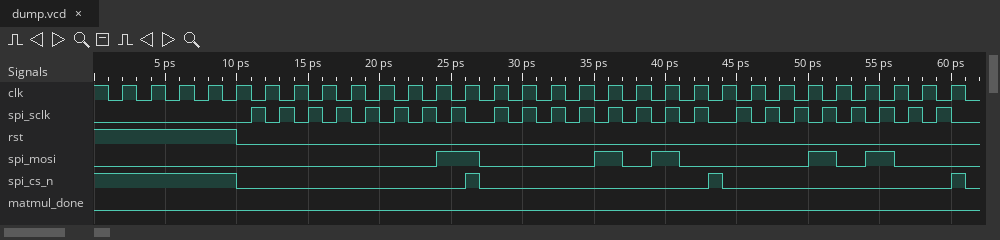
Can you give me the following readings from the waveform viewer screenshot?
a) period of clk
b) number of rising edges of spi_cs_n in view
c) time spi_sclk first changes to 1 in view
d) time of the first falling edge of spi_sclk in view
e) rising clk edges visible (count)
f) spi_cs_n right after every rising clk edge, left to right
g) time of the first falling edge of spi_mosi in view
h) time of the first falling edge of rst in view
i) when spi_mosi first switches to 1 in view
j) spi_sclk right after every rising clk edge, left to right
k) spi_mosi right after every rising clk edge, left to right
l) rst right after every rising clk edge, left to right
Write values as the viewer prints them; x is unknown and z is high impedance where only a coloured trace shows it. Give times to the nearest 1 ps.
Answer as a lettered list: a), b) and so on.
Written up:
a) 2 ps
b) 3
c) 11 ps
d) 12 ps
e) 30
f) 1 1 1 1 0 0 0 0 0 0 0 0 1 0 0 0 0 0 0 0 0 0 0 0 0 0 0 0 0 1
g) 27 ps
h) 10 ps
i) 24 ps
j) 0 0 0 0 0 0 0 0 0 0 0 0 0 1 1 1 1 1 1 1 1 0 0 0 0 0 0 0 0 0
k) 0 0 0 0 0 0 0 0 0 0 0 1 1 0 0 0 0 1 0 1 0 0 0 0 1 0 1 0 0 0
l) 1 1 1 1 0 0 0 0 0 0 0 0 0 0 0 0 0 0 0 0 0 0 0 0 0 0 0 0 0 0
